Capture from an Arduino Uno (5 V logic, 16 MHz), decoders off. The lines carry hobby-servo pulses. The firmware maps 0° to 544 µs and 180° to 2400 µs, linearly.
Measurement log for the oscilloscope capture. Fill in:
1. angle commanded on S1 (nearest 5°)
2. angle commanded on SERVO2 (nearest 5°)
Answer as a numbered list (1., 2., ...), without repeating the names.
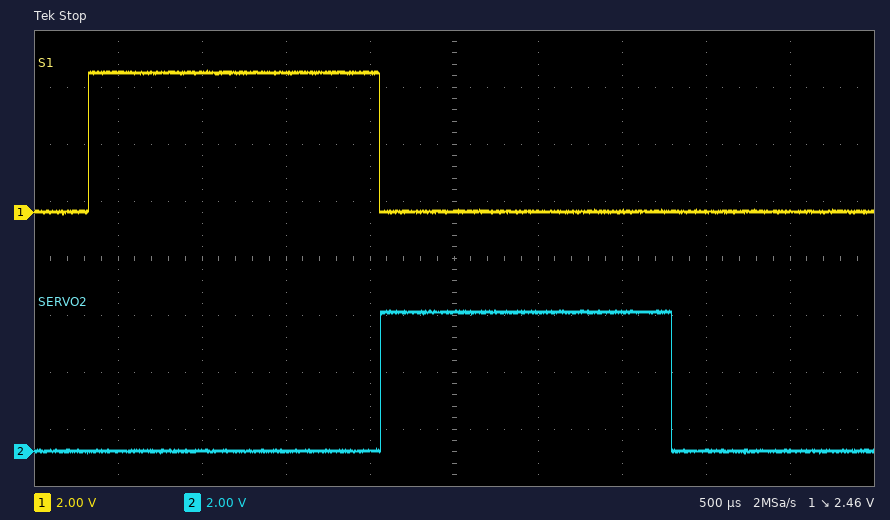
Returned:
1. 115°
2. 115°
